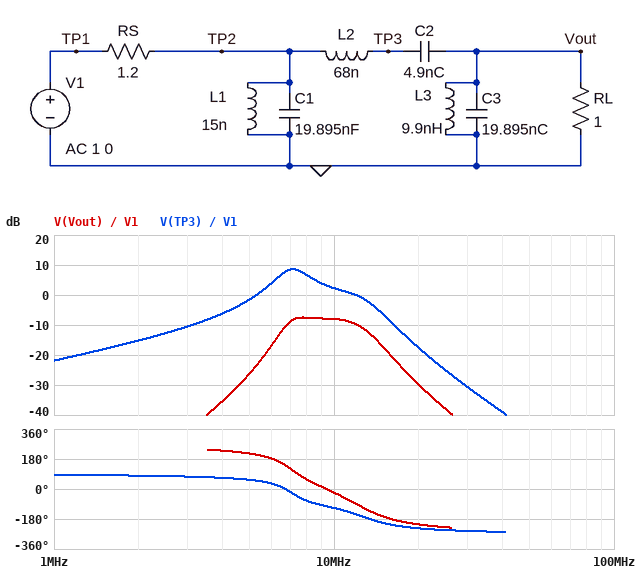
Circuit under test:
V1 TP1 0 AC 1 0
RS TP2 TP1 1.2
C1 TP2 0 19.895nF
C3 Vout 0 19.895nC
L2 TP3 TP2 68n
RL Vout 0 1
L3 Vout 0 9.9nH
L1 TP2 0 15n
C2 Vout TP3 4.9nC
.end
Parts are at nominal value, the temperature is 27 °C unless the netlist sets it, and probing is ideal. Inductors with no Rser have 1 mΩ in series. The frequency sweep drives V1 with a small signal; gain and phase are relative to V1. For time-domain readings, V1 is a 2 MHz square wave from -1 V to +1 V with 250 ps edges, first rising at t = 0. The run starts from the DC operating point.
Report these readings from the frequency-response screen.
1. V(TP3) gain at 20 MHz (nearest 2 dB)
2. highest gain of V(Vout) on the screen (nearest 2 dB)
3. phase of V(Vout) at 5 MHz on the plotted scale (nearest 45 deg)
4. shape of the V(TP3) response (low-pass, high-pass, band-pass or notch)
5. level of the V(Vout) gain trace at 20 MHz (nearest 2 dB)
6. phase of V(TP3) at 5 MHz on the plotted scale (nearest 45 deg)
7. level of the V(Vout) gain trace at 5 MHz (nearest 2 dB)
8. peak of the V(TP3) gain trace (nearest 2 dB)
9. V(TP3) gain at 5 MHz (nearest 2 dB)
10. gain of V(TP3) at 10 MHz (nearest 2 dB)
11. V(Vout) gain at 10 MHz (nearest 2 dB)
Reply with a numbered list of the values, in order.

1. -18 dB
2. -8 dB
3. 225 deg
4. band-pass
5. -30 dB
6. 45 deg
7. -26 dB
8. 8 dB
9. -2 dB
10. 2 dB
11. -8 dB
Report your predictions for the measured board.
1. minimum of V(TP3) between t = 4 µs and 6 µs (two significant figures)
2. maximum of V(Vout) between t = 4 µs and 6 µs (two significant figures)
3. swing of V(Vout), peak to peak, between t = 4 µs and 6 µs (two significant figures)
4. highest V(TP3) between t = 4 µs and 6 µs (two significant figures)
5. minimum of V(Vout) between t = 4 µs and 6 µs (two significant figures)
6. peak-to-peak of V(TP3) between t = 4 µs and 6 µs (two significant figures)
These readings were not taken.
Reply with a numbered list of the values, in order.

1. -1.1 V
2. 180 mV
3. 360 mV
4. 1.1 V
5. -180 mV
6. 2.2 V
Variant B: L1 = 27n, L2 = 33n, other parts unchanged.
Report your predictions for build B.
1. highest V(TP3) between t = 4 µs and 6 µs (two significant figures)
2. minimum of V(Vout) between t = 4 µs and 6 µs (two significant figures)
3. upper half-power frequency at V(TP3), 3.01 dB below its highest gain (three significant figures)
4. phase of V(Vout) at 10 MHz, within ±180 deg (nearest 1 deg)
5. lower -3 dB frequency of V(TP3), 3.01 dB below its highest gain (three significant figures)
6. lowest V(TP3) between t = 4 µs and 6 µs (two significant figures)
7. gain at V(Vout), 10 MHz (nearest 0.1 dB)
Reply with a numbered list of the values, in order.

1. 1.6 V
2. -240 mV
3. 17.2 MHz
4. 23 deg
5. 4.90 MHz
6. -1.6 V
7. -9.4 dB
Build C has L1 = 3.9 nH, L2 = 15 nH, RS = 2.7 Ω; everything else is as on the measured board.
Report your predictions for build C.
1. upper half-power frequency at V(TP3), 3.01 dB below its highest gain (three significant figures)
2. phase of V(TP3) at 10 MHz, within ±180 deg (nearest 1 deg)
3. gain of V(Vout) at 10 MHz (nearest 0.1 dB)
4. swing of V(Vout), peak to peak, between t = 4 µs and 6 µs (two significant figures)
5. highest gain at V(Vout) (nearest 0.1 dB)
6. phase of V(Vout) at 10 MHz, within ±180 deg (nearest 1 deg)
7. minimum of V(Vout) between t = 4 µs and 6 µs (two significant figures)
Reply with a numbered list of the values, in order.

1. 25.8 MHz
2. 69 deg
3. -23.8 dB
4. 220 mV
5. -10.4 dB
6. 162 deg
7. -110 mV
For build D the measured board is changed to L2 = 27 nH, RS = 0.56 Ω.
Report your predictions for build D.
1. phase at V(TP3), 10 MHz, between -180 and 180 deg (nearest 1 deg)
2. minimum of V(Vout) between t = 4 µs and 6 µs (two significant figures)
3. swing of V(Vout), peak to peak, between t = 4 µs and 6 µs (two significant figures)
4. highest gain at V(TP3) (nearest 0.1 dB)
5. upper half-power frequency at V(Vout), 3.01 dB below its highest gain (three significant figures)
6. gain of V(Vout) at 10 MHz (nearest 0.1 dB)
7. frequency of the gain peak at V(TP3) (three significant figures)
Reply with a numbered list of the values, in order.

1. -37 deg
2. -360 mV
3. 710 mV
4. 7.8 dB
5. 18.5 MHz
6. -6.3 dB
7. 16.6 MHz
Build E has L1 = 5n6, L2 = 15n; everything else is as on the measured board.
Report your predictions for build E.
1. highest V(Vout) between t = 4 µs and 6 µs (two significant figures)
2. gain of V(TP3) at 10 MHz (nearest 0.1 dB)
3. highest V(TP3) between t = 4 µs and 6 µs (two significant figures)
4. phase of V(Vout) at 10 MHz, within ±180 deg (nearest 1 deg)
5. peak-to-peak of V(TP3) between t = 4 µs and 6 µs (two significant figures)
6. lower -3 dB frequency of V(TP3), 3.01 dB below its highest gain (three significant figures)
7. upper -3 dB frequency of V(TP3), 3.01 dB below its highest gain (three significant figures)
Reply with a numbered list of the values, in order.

1. 230 mV
2. -2.5 dB
3. 940 mV
4. 134 deg
5. 1.9 V
6. 21.1 MHz
7. 25.2 MHz
